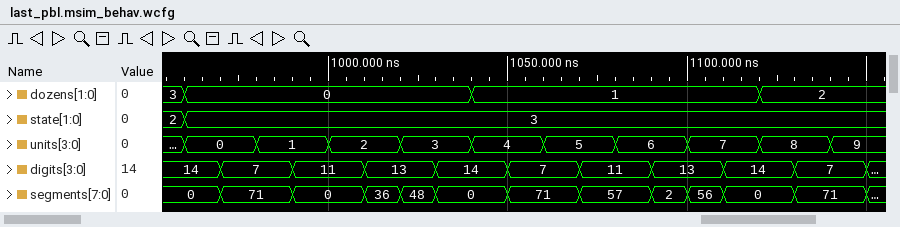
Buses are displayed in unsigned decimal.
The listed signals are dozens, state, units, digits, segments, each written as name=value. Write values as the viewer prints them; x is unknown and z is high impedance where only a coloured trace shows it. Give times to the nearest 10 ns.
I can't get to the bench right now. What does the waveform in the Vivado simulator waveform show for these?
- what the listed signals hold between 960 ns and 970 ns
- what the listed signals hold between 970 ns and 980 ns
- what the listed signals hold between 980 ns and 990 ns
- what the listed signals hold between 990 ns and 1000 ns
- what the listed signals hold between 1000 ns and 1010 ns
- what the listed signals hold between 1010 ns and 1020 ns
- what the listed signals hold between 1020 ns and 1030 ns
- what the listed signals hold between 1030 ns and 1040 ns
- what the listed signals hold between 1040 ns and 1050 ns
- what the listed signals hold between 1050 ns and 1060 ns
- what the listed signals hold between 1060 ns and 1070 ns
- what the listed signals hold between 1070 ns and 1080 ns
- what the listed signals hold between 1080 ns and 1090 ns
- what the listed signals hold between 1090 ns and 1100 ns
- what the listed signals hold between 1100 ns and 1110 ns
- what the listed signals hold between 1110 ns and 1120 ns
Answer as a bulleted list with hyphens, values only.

- dozens=0, state=3, units=0, digits=14, segments=0
- dozens=0, state=3, units=0, digits=7, segments=71
- dozens=0, state=3, units=1, digits=7, segments=71
- dozens=0, state=3, units=1, digits=11, segments=0
- dozens=0, state=3, units=2, digits=11, segments=0
- dozens=0, state=3, units=2, digits=13, segments=36
- dozens=0, state=3, units=3, digits=13, segments=48
- dozens=0, state=3, units=3, digits=14, segments=0
- dozens=1, state=3, units=4, digits=14, segments=0
- dozens=1, state=3, units=4, digits=7, segments=71
- dozens=1, state=3, units=5, digits=7, segments=71
- dozens=1, state=3, units=5, digits=11, segments=57
- dozens=1, state=3, units=6, digits=11, segments=57
- dozens=1, state=3, units=6, digits=13, segments=2
- dozens=1, state=3, units=7, digits=13, segments=56
- dozens=1, state=3, units=7, digits=14, segments=0
